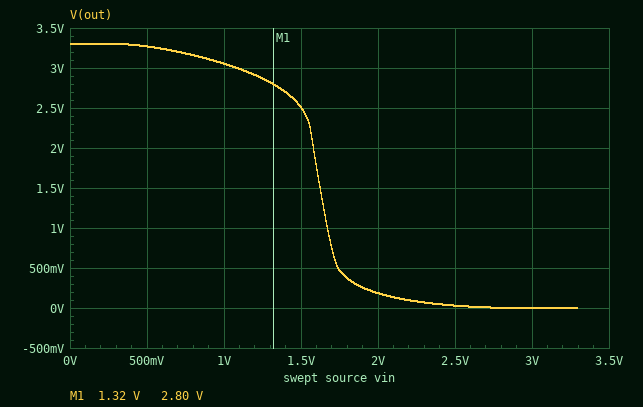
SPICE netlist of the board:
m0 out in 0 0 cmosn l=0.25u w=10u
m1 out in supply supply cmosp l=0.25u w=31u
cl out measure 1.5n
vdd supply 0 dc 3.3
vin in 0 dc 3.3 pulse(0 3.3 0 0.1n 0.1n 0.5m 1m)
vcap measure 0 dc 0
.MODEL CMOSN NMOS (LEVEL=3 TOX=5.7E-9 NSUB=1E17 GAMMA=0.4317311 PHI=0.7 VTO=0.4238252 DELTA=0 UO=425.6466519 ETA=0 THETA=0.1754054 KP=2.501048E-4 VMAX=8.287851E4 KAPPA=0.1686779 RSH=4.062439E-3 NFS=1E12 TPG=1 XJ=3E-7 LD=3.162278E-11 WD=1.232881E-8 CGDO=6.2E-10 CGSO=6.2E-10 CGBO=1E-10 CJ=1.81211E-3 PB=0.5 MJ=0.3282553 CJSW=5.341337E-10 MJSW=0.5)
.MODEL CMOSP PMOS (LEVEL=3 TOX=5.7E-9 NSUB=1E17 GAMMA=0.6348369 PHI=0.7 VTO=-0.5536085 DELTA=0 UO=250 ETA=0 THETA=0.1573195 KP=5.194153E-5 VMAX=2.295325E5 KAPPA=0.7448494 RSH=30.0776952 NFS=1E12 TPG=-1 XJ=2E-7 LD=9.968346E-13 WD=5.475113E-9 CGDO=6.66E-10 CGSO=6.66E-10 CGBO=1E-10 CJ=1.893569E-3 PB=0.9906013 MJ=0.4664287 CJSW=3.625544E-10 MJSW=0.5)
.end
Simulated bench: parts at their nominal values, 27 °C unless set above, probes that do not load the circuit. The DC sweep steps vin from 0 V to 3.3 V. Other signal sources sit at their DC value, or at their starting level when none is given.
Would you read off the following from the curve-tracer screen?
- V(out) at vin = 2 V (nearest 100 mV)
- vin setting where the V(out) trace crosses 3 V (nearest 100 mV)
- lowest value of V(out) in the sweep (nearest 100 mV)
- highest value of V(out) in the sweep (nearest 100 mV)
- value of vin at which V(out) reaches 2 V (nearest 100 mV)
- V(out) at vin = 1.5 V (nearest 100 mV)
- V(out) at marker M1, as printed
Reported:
200 mV
1.1 V
0 V
3.3 V
1.6 V
2.5 V
2.80 V
